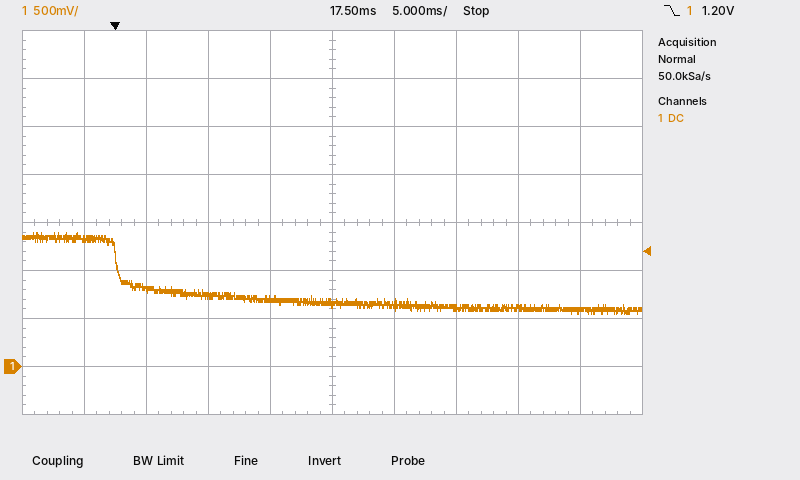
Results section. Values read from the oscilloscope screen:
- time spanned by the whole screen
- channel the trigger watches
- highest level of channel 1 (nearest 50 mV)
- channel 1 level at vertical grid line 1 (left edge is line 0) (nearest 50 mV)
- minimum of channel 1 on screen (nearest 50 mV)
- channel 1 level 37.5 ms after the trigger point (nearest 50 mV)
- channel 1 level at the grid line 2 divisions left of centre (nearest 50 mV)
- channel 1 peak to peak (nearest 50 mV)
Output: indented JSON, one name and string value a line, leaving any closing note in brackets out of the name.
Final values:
{
  "time spanned by the whole screen": "50 ms",
  "channel the trigger watches": "channel 1",
  "highest level of channel 1": "1.40 V",
  "channel 1 level at vertical grid line 1 (left edge is line 0)": "1.35 V",
  "minimum of channel 1 on screen": "550 mV",
  "channel 1 level 37.5 ms after the trigger point": "600 mV",
  "channel 1 level at the grid line 2 divisions left of centre": "750 mV",
  "channel 1 peak to peak": "850 mV"
}
